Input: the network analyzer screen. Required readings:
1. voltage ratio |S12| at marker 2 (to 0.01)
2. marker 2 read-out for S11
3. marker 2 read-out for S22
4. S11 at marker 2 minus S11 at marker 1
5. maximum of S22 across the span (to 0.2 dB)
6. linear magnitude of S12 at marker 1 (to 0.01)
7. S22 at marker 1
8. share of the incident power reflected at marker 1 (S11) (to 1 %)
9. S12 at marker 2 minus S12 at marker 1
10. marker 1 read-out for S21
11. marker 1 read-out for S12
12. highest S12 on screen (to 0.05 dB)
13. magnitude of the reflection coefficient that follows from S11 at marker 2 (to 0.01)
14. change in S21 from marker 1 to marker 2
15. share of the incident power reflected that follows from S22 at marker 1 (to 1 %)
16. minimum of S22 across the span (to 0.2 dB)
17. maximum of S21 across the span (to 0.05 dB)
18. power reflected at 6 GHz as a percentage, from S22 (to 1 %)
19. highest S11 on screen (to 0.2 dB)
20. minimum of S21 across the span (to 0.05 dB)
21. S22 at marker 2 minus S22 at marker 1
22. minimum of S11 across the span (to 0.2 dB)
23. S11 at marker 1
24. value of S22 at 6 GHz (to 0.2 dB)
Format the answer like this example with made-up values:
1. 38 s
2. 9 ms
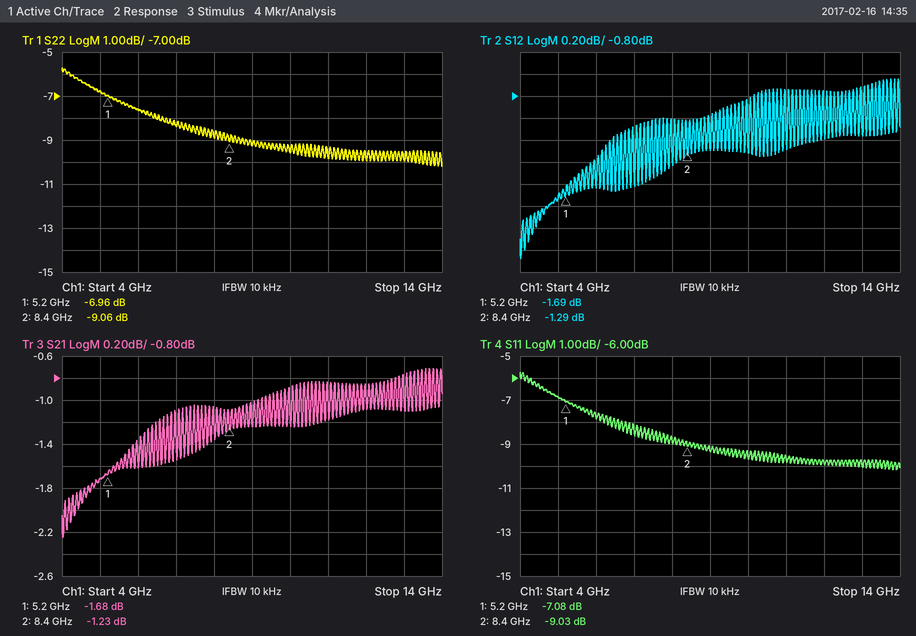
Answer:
1. 0.86
2. -9.03 dB
3. -9.06 dB
4. -1.95 dB
5. -5.8 dB
6. 0.82
7. -6.96 dB
8. 20 %
9. 0.40 dB
10. -1.68 dB
11. -1.69 dB
12. -0.65 dB
13. 0.35
14. 0.45 dB
15. 20 %
16. -10.2 dB
17. -0.70 dB
18. 17 %
19. -5.8 dB
20. -2.25 dB
21. -2.10 dB
22. -10.2 dB
23. -7.08 dB
24. -7.6 dB
